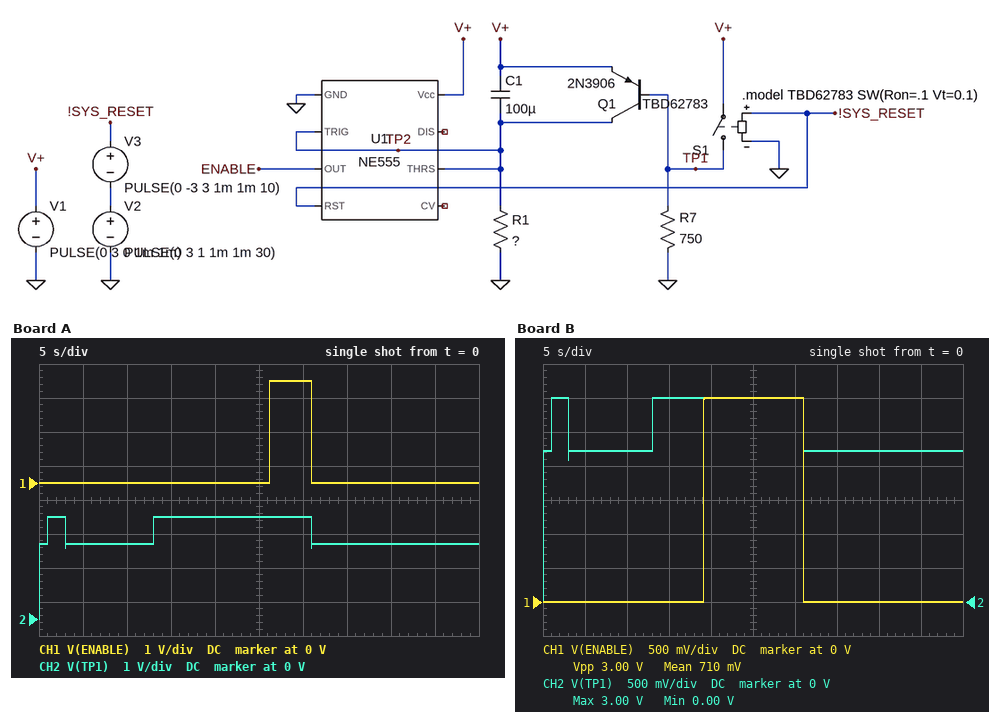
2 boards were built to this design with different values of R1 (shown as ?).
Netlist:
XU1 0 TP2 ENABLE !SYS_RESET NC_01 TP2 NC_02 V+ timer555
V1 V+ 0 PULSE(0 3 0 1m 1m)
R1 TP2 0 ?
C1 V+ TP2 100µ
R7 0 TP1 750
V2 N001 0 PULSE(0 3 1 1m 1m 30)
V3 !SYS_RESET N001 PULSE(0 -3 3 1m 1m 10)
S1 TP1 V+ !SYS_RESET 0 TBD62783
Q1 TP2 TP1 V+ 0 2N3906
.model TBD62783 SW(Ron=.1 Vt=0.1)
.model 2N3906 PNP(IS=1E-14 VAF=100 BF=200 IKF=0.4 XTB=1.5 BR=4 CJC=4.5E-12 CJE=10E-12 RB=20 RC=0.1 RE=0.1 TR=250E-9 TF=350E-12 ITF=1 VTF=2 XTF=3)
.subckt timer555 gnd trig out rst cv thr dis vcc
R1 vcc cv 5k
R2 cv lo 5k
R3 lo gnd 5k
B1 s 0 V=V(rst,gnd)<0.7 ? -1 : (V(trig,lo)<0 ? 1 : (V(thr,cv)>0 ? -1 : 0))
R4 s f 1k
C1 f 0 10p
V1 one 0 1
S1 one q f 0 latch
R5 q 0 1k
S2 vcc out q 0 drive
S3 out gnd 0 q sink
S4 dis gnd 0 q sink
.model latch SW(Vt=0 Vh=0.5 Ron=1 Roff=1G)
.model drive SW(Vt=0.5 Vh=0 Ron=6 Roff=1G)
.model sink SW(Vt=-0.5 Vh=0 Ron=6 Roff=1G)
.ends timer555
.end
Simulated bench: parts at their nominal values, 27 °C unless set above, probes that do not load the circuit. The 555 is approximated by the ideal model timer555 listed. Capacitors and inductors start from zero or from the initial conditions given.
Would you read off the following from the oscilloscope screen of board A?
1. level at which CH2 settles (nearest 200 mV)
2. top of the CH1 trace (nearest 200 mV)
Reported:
2.2 V
3.0 V
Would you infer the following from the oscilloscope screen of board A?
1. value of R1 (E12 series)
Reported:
120 kΩ
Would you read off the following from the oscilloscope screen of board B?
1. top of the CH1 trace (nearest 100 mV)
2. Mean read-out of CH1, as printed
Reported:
3.0 V
710 mV
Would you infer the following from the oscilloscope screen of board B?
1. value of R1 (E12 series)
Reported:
56 kΩ
